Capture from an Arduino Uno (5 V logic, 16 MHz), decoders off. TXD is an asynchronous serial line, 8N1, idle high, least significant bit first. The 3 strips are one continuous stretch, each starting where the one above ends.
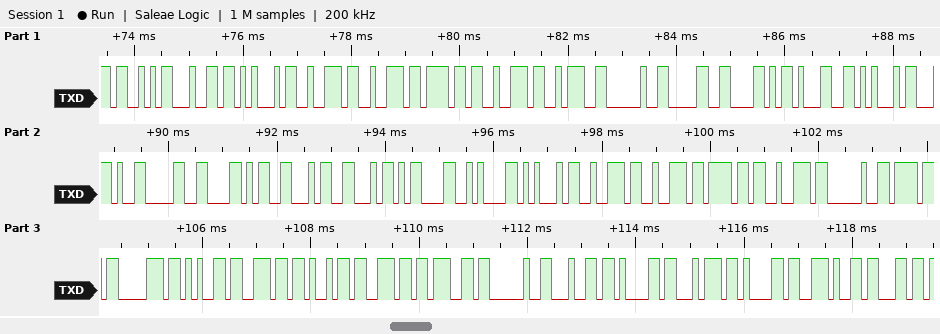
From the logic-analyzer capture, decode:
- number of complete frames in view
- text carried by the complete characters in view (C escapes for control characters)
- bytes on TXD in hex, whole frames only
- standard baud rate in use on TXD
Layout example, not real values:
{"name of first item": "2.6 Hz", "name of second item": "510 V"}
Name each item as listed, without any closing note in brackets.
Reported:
{"number of complete frames in view": "40", "text carried by the complete characters in view": "\"SdError: 0X1E,0XFF\\r\\nError opening data.c\"", "bytes on TXD in hex, whole frames only": "53 64 45 72 72 6F 72 3A 20 30 58 31 45 2C 30 58 46 46 0D 0A 45 72 72 6F 72 20 6F 70 65 6E 69 6E 67 20 64 61 74 61 2E 63", "standard baud rate in use on TXD": "9600 baud"}
